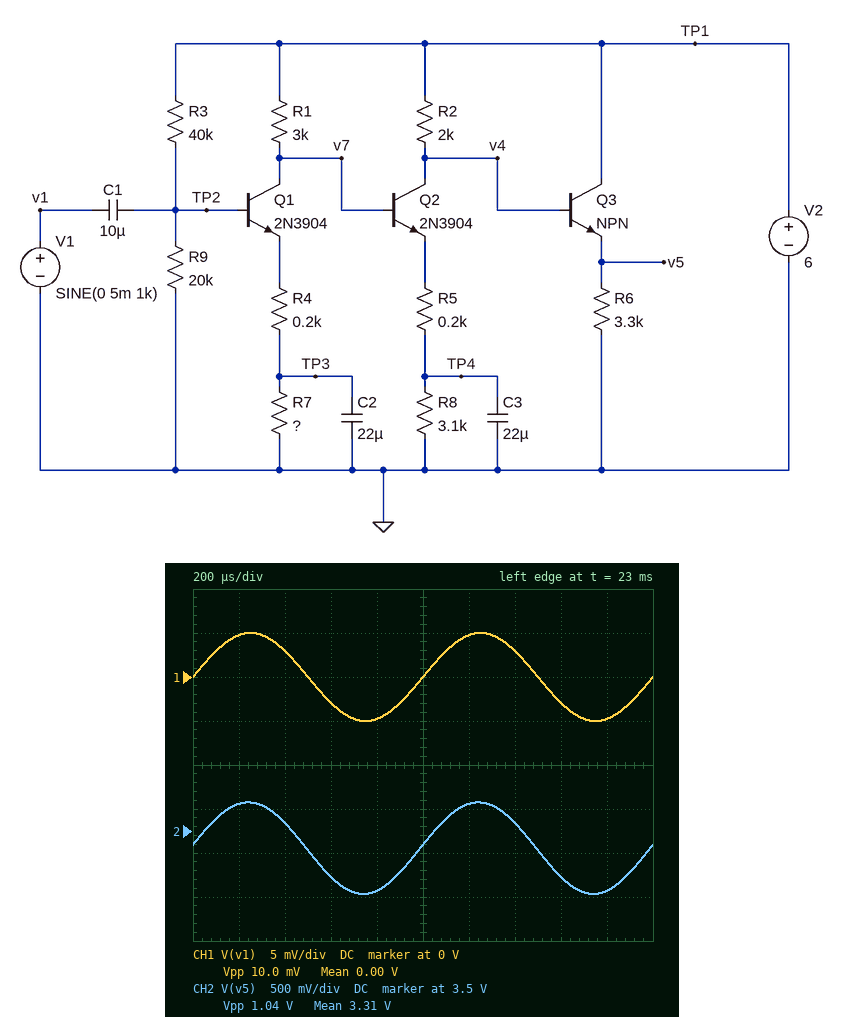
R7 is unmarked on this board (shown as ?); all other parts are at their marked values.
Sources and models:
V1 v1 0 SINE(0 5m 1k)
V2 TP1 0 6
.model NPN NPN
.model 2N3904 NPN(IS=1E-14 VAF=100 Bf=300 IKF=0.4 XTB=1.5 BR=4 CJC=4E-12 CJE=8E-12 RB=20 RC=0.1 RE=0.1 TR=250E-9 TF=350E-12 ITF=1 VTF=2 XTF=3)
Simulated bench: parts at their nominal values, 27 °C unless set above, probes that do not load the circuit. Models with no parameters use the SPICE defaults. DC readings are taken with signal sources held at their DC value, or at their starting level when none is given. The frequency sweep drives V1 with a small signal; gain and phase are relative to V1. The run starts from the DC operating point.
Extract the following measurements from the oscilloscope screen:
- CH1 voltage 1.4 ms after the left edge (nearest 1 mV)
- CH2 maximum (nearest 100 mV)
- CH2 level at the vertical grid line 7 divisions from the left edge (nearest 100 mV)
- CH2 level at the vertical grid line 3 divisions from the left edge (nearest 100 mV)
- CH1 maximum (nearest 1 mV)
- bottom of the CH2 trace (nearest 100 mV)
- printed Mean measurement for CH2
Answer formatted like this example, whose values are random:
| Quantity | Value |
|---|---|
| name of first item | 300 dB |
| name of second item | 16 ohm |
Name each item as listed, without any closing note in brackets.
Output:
| Quantity | Value |
|---|---|
| CH1 voltage 1.4 ms after the left edge | 3 mV |
| CH2 maximum | 3.8 V |
| CH2 level at the vertical grid line 7 divisions from the left edge | 3.6 V |
| CH2 level at the vertical grid line 3 divisions from the left edge | 3.0 V |
| CH1 maximum | 5 mV |
| bottom of the CH2 trace | 2.8 V |
| printed Mean measurement for CH2 | 3.31 V |
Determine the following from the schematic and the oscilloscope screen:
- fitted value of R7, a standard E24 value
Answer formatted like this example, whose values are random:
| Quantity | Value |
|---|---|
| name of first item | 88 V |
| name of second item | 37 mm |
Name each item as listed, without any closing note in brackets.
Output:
| Quantity | Value |
|---|---|
| fitted value of R7, a standard E24 value | 1.6 kΩ |
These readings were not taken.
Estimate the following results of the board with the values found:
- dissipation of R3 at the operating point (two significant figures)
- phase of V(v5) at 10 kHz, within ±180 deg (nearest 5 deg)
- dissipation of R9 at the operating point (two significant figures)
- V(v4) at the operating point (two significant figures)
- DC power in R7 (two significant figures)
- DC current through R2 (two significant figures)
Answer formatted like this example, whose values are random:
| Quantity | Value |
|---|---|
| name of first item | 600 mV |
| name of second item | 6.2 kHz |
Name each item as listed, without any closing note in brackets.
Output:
| Quantity | Value |
|---|---|
| dissipation of R3 at the operating point | 410 µW |
| phase of V(v5) at 10 kHz, within ±180 deg | 0 deg |
| dissipation of R9 at the operating point | 190 µW |
| V(v4) at the operating point | 4.1 V |
| DC power in R7 | 860 µW |
| DC current through R2 | 960 µA |
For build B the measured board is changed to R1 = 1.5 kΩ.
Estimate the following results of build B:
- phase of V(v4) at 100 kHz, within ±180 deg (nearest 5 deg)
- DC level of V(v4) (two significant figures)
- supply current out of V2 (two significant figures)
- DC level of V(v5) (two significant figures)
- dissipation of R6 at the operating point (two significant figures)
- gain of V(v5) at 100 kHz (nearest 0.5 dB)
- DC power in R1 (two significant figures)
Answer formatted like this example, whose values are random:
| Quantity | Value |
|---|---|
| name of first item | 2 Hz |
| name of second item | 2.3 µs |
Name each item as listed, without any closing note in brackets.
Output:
| Quantity | Value |
|---|---|
| phase of V(v4) at 100 kHz, within ±180 deg | -165 deg |
| DC level of V(v4) | 4.0 V |
| supply current out of V2 | 3.0 mA |
| DC level of V(v5) | 3.2 V |
| dissipation of R6 at the operating point | 3.1 mW |
| gain of V(v5) at 100 kHz | -6.0 dB |
| DC power in R1 | 1.3 mW |
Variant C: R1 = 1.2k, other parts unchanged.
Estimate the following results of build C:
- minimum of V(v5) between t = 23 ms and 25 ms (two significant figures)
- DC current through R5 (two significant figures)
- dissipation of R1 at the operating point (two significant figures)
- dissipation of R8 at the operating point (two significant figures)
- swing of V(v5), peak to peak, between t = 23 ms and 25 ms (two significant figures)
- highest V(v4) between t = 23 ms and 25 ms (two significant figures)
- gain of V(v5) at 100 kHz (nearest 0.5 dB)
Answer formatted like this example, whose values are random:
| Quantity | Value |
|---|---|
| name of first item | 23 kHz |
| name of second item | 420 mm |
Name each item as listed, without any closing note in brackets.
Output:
| Quantity | Value |
|---|---|
| minimum of V(v5) between t = 23 ms and 25 ms | 3.3 V |
| DC current through R5 | 1.2 mA |
| dissipation of R1 at the operating point | 1.3 mW |
| dissipation of R8 at the operating point | 4.7 mW |
| swing of V(v5), peak to peak, between t = 23 ms and 25 ms | 5.2 mV |
| highest V(v4) between t = 23 ms and 25 ms | 4.1 V |
| gain of V(v5) at 100 kHz | -5.0 dB |
